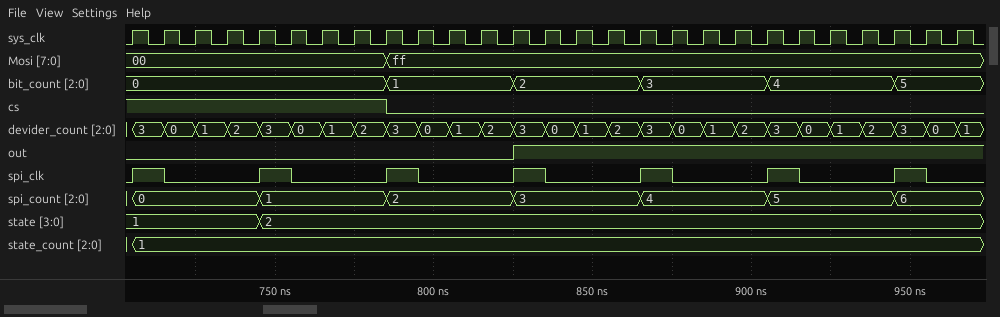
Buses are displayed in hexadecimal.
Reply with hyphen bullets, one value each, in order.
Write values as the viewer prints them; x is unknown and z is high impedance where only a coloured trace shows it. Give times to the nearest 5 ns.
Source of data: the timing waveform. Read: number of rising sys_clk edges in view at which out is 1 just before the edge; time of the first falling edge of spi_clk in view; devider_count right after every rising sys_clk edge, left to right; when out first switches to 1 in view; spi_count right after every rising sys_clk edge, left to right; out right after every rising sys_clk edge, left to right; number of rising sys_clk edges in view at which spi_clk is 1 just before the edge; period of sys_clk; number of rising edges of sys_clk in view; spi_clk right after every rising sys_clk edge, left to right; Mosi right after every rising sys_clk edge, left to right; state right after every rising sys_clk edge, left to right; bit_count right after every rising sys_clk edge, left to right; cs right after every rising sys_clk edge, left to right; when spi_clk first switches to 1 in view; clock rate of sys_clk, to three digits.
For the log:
- 14
- 715 ns
- 3, 0, 1, 2, 3, 0, 1, 2, 3, 0, 1, 2, 3, 0, 1, 2, 3, 0, 1, 2, 3, 0, 1, 2, 3, 0, 1
- 825 ns
- 0, 0, 0, 0, 1, 1, 1, 1, 2, 2, 2, 2, 3, 3, 3, 3, 4, 4, 4, 4, 5, 5, 5, 5, 6, 6, 6
- 0 0 0 0 0 0 0 0 0 0 0 0 1 1 1 1 1 1 1 1 1 1 1 1 1 1 1
- 7
- 10 ns
- 27
- 1 0 0 0 1 0 0 0 1 0 0 0 1 0 0 0 1 0 0 0 1 0 0 0 1 0 0
- 00, 00, 00, 00, 00, 00, 00, 00, ff, ff, ff, ff, ff, ff, ff, ff, ff, ff, ff, ff, ff, ff, ff, ff, ff, ff, ff
- 1, 1, 1, 1, 2, 2, 2, 2, 2, 2, 2, 2, 2, 2, 2, 2, 2, 2, 2, 2, 2, 2, 2, 2, 2, 2, 2
- 0, 0, 0, 0, 0, 0, 0, 0, 1, 1, 1, 1, 2, 2, 2, 2, 3, 3, 3, 3, 4, 4, 4, 4, 5, 5, 5
- 1 1 1 1 1 1 1 1 0 0 0 0 0 0 0 0 0 0 0 0 0 0 0 0 0 0 0
- 705 ns
- 100 MHz
